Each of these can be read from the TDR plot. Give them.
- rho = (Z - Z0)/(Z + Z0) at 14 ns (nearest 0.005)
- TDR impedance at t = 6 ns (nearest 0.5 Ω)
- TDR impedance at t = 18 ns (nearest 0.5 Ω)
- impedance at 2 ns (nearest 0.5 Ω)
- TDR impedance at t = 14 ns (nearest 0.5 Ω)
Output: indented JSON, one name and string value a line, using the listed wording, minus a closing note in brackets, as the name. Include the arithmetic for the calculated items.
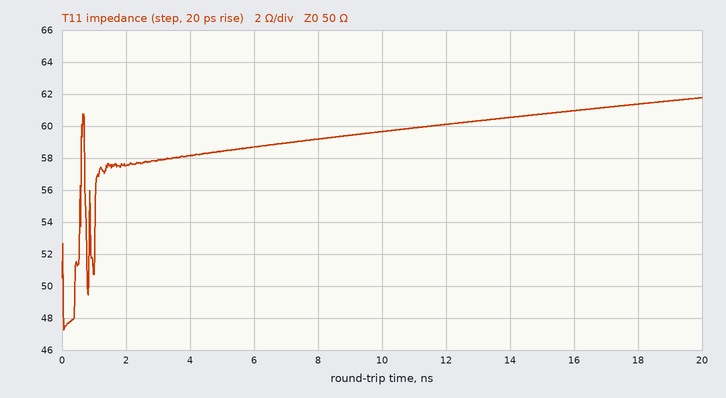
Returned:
{
  "rho = (Z - Z0)/(Z + Z0) at 14 ns": "(60.5 − 50)/(60.5 + 50) ≈ +0.095",
  "TDR impedance at t = 6 ns": "58.5 Ω",
  "TDR impedance at t = 18 ns": "61.5 Ω",
  "impedance at 2 ns": "57.5 Ω",
  "TDR impedance at t = 14 ns": "60.5 Ω"
}
